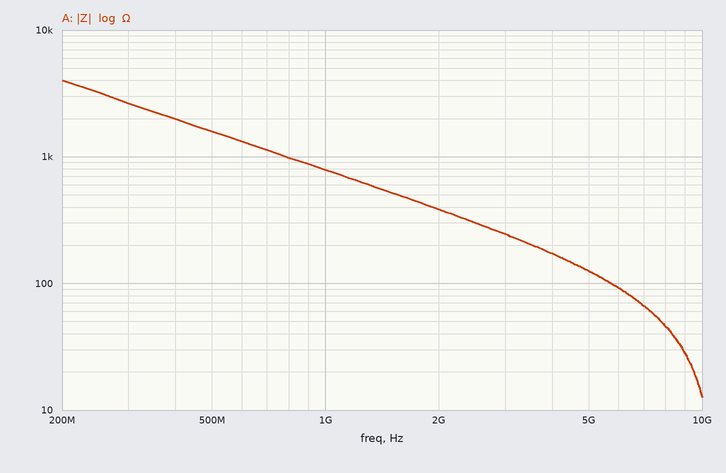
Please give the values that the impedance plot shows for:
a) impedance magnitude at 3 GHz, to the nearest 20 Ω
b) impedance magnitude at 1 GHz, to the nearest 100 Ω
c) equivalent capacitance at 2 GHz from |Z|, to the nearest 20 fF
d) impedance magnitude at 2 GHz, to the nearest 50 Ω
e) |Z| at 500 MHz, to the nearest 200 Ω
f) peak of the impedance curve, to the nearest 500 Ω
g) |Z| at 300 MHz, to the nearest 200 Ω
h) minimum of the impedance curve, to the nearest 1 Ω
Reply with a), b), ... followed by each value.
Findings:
a) 240 Ω
b) 800 Ω
c) 200 fF
d) 400 Ω
e) 1.6 kΩ
f) 4.0 kΩ
g) 2.6 kΩ
h) 13 Ω
